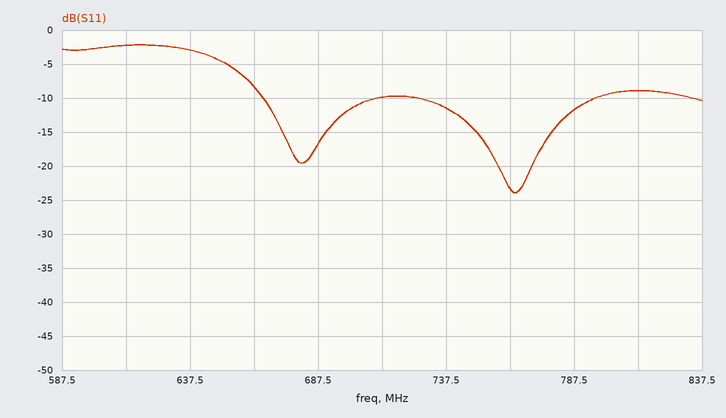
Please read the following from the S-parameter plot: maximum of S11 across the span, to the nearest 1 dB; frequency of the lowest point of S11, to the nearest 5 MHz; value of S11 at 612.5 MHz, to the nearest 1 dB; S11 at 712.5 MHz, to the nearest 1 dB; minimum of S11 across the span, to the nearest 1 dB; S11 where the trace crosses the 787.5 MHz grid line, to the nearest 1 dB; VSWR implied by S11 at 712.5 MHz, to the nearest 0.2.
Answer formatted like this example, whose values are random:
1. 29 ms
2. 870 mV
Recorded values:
1. -2 dB
2. 765 MHz
3. -2 dB
4. -10 dB
5. -24 dB
6. -12 dB
7. 2.0
